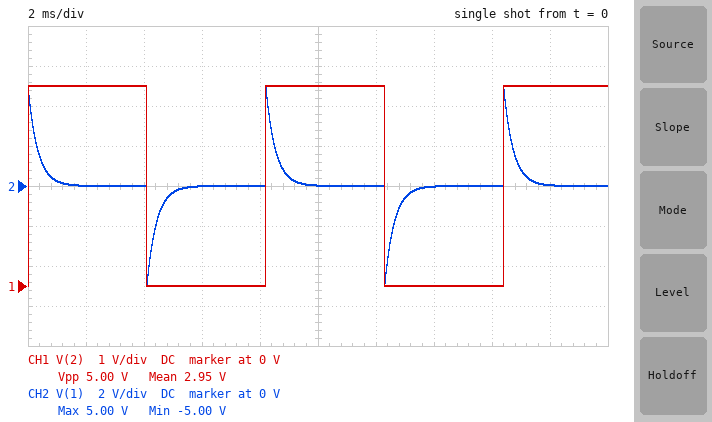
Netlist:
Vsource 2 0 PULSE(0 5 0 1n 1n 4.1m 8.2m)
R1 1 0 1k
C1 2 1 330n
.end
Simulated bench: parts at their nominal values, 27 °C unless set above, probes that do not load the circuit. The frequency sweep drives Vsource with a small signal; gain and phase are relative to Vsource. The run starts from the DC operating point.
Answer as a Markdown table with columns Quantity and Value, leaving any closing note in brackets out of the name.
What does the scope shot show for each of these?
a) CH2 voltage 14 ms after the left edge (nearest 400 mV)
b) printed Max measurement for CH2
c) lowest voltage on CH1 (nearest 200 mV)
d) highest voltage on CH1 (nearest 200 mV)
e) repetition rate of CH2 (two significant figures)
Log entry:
| Quantity | Value |
|---|---|
| CH2 voltage 14 ms after the left edge | 0 V |
| printed Max measurement for CH2 | 5.00 V |
| lowest voltage on CH1 | 0 V |
| highest voltage on CH1 | 5.0 V |
| repetition rate of CH2 | 120 Hz |
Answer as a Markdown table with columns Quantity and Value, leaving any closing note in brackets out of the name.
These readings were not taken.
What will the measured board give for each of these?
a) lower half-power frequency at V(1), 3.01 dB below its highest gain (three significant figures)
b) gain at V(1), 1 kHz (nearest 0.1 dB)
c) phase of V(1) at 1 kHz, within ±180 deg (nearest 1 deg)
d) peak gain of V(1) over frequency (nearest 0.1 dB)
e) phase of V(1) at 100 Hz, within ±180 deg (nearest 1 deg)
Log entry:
| Quantity | Value |
|---|---|
| lower half-power frequency at V(1), 3.01 dB below its highest gain | 482 Hz |
| gain at V(1), 1 kHz | -0.9 dB |
| phase of V(1) at 1 kHz, within ±180 deg | 26 deg |
| peak gain of V(1) over frequency | 0 dB |
| phase of V(1) at 100 Hz, within ±180 deg | 78 deg |
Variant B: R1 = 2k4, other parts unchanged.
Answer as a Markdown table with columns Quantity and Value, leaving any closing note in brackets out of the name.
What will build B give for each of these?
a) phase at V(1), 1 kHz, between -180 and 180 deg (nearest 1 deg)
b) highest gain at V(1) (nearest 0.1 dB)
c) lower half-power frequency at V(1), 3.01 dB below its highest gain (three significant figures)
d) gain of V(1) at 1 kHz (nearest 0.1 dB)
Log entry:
| Quantity | Value |
|---|---|
| phase at V(1), 1 kHz, between -180 and 180 deg | 11 deg |
| highest gain at V(1) | 0 dB |
| lower half-power frequency at V(1), 3.01 dB below its highest gain | 201 Hz |
| gain of V(1) at 1 kHz | -0.2 dB |
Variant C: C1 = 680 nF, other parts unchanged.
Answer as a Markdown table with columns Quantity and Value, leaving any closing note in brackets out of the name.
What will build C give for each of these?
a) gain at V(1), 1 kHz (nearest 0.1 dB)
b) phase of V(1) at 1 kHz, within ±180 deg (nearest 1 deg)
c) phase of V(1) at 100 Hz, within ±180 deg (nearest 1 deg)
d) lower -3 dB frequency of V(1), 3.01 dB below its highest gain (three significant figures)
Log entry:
| Quantity | Value |
|---|---|
| gain at V(1), 1 kHz | -0.2 dB |
| phase of V(1) at 1 kHz, within ±180 deg | 13 deg |
| phase of V(1) at 100 Hz, within ±180 deg | 67 deg |
| lower -3 dB frequency of V(1), 3.01 dB below its highest gain | 234 Hz |
